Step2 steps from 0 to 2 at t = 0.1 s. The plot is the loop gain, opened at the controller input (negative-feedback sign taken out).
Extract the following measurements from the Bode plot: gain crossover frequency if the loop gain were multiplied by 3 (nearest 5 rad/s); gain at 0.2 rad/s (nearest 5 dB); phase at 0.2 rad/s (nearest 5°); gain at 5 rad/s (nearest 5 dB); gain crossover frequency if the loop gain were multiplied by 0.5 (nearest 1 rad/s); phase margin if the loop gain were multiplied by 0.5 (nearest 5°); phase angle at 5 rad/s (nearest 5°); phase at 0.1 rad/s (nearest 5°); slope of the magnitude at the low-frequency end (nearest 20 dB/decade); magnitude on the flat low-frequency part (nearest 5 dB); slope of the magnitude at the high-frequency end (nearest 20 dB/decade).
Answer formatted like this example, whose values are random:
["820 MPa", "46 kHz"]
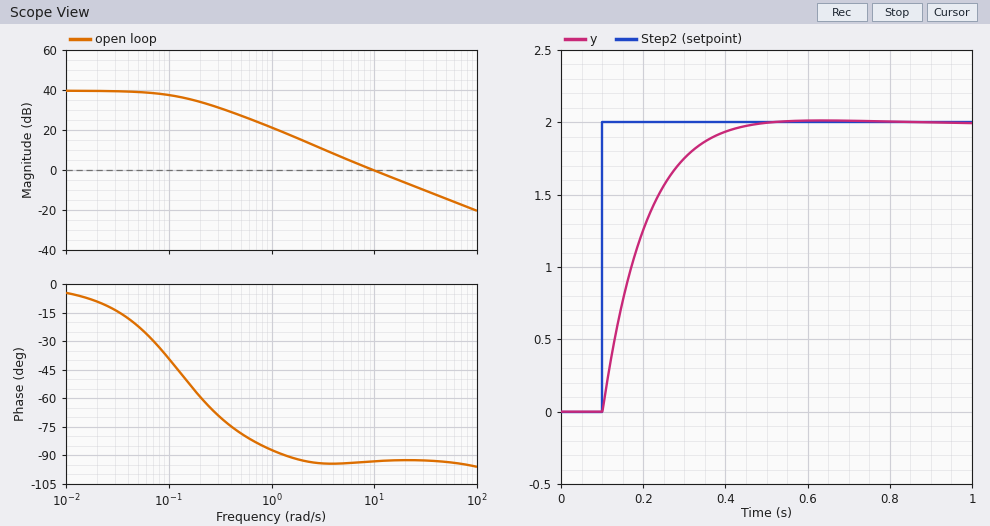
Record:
["30 rad/s", "35 dB", "-60°", "5 dB", "5 rad/s", "85°", "-95°", "-40°", "0 dB/decade", "40 dB", "-20 dB/decade"]
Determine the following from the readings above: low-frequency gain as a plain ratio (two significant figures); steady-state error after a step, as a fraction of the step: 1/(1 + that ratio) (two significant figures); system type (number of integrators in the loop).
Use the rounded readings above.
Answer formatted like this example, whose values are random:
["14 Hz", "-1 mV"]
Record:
["100", "0.0099", "0"]
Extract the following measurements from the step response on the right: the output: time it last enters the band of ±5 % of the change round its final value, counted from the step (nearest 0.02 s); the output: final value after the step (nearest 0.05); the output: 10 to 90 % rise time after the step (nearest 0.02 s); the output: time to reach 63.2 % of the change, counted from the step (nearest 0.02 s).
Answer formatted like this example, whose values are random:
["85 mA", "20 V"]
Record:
["0.26 s", "2.00", "0.20 s", "0.10 s"]
